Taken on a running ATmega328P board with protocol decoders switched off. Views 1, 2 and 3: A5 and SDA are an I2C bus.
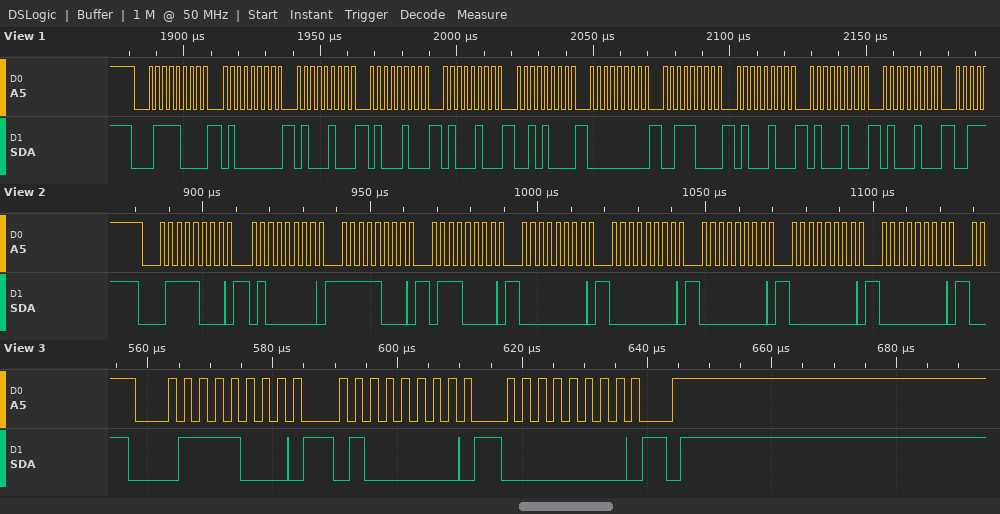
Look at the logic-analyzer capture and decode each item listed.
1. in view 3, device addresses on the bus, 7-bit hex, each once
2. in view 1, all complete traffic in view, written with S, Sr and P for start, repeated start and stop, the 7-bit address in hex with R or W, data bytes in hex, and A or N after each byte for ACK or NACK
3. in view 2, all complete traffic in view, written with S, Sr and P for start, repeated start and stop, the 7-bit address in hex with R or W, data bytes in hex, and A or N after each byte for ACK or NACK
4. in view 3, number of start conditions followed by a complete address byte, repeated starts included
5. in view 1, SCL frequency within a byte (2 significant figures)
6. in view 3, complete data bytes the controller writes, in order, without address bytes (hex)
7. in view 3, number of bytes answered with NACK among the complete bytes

0x3C
S 3CW A 40 A 44 A 44 A 44 A 28 A 00 A 38 A 44 A 44 A 44 A
S 3CW A 40 A F8 A 70 A 00 A 00 A 00 A 00 A 00 A
1
400 kHz
40 00
0
